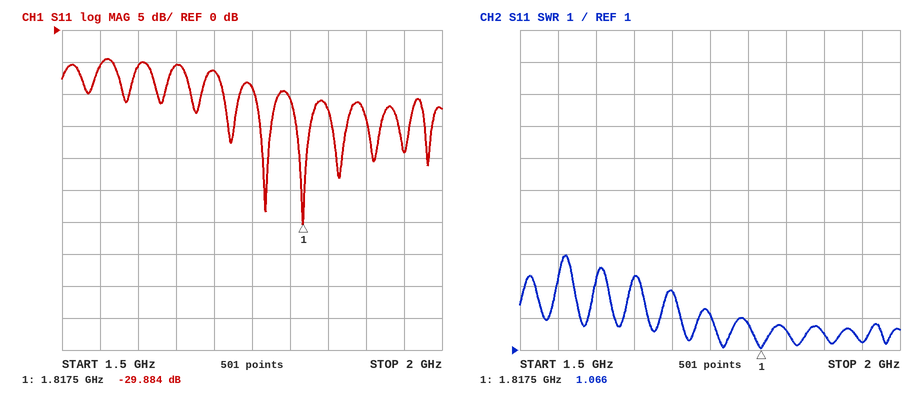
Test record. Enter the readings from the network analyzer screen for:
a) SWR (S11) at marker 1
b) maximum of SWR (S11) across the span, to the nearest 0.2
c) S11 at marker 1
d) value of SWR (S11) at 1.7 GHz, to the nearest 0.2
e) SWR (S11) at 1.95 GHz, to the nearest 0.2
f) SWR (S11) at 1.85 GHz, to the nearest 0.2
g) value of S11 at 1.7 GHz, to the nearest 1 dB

1.066
4.0
-29.884 dB
2.8
1.2
1.6
-6 dB
